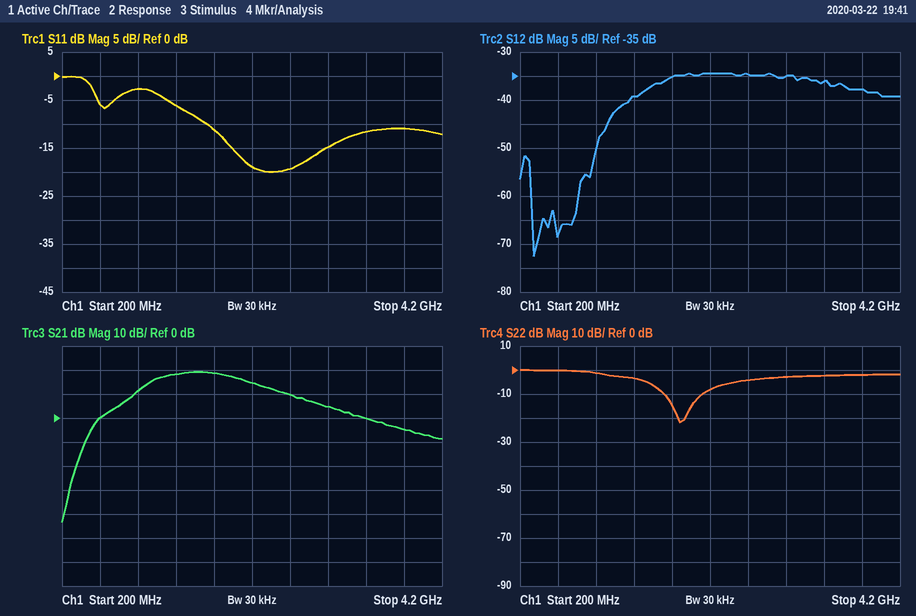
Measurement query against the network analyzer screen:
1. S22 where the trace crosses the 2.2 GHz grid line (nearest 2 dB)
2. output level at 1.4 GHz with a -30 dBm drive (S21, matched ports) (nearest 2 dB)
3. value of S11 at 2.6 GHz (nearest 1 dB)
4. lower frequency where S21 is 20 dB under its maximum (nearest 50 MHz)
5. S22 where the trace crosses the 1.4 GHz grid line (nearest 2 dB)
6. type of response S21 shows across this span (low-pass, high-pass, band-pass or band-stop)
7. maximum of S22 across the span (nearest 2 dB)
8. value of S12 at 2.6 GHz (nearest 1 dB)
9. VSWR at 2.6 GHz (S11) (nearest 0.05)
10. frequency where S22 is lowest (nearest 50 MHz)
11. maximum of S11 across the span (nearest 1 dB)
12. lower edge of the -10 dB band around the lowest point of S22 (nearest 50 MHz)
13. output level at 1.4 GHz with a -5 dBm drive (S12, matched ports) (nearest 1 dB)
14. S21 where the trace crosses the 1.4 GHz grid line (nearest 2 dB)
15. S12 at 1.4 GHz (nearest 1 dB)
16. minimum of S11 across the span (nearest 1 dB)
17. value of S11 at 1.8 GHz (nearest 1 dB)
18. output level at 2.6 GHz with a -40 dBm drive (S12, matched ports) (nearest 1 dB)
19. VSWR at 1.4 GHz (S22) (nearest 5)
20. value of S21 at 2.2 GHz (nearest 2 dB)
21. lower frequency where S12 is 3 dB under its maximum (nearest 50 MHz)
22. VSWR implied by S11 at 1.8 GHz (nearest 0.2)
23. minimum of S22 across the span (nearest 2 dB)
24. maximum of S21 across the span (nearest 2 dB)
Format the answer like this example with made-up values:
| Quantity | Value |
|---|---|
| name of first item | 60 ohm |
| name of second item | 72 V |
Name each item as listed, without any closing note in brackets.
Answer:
| Quantity | Value |
|---|---|
| S22 where the trace crosses the 2.2 GHz grid line | -8 dB |
| output level at 1.4 GHz with a -30 dBm drive (S21, matched ports) | -12 dBm |
| value of S11 at 2.6 GHz | -19 dB |
| lower frequency where S21 is 20 dB under its maximum | 600 MHz |
| S22 where the trace crosses the 1.4 GHz grid line | -4 dB |
| type of response S21 shows across this span | band-pass |
| maximum of S22 across the span | 0 dB |
| value of S12 at 2.6 GHz | -35 dB |
| VSWR at 2.6 GHz (S11) | 1.25 |
| frequency where S22 is lowest | 1.90 GHz |
| maximum of S11 across the span | 0 dB |
| lower edge of the -10 dB band around the lowest point of S22 | 1.70 GHz |
| output level at 1.4 GHz with a -5 dBm drive (S12, matched ports) | -44 dBm |
| S21 where the trace crosses the 1.4 GHz grid line | 18 dB |
| S12 at 1.4 GHz | -39 dB |
| minimum of S11 across the span | -20 dB |
| value of S11 at 1.8 GHz | -11 dB |
| output level at 2.6 GHz with a -40 dBm drive (S12, matched ports) | -75 dBm |
| VSWR at 1.4 GHz (S22) | 5 |
| value of S21 at 2.2 GHz | 14 dB |
| lower frequency where S12 is 3 dB under its maximum | 1.55 GHz |
| VSWR implied by S11 at 1.8 GHz | 1.8 |
| minimum of S22 across the span | -22 dB |
| maximum of S21 across the span | 20 dB |
